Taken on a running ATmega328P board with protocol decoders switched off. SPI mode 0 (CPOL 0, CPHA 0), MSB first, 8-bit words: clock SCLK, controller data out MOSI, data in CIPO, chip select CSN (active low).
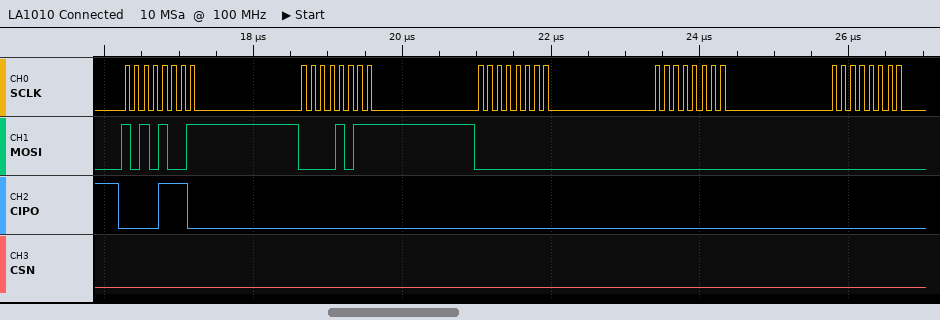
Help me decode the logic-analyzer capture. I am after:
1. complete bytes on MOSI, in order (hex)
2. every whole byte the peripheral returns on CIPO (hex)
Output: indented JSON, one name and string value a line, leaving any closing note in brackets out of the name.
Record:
{
  "complete bytes on MOSI, in order": "A9 0B 00 00 00",
  "every whole byte the peripheral returns on CIPO": "0E 00 00 00 00"
}
